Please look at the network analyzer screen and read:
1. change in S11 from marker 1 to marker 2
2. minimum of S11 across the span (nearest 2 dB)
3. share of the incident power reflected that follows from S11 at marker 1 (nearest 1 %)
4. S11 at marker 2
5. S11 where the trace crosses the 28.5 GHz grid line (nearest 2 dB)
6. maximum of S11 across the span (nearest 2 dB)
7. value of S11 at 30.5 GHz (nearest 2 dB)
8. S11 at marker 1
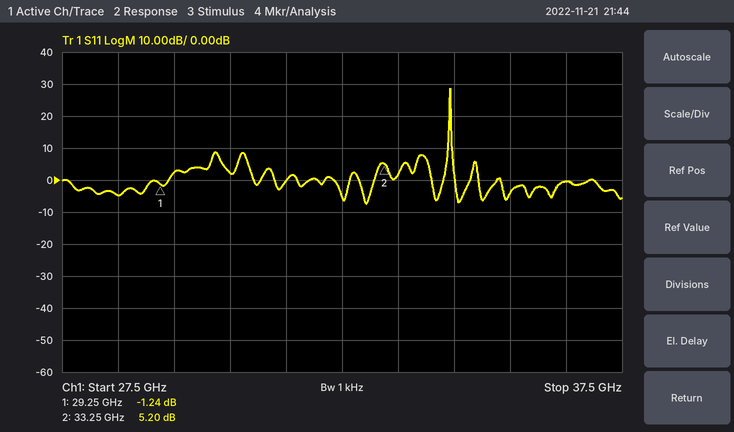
6.44 dB
-8 dB
75 %
5.20 dB
-4 dB
28 dB
2 dB
-1.24 dB
